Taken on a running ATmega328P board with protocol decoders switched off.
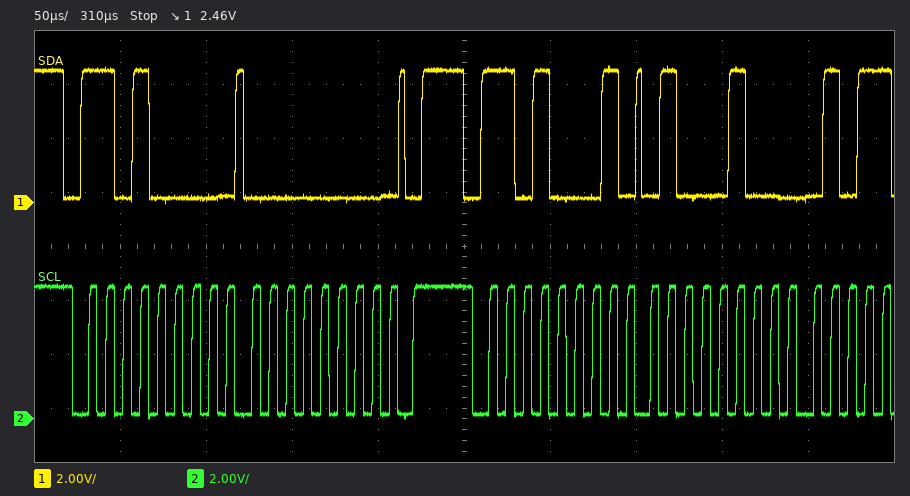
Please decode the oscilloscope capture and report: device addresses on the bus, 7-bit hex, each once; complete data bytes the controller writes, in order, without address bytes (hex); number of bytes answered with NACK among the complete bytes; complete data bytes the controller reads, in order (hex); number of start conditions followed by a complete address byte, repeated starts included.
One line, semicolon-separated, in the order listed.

0x68; 00; 0; 44; 2
